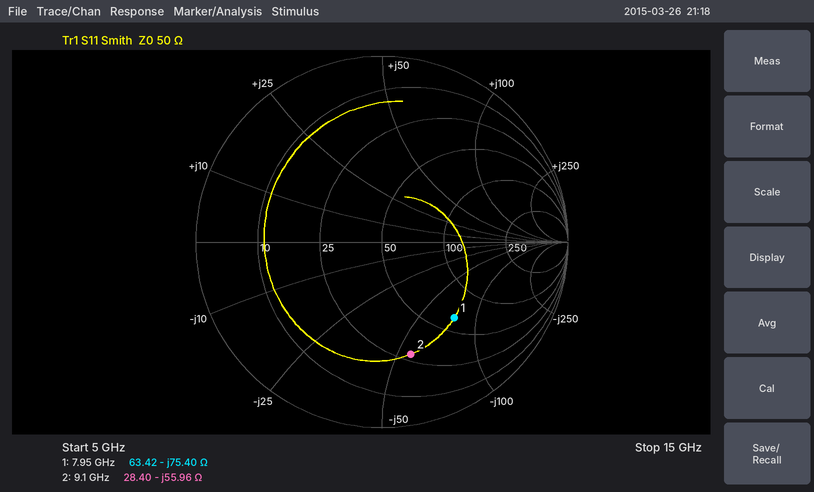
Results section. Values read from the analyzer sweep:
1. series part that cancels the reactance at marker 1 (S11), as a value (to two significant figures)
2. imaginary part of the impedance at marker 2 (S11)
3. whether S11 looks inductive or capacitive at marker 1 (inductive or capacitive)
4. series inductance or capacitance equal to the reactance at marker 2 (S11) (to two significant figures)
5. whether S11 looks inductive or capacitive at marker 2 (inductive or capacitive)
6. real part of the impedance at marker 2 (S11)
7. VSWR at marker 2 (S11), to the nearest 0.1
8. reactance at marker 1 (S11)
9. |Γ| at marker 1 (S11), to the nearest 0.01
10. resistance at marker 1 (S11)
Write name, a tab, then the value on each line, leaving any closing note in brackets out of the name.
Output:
series part that cancels the reactance at marker 1 (S11), as a value	1.5 nH
imaginary part of the impedance at marker 2	-55.96 Ω
whether S11 looks inductive or capacitive at marker 1	capacitive
series inductance or capacitance equal to the reactance at marker 2 (S11)	310 fF
whether S11 looks inductive or capacitive at marker 2	capacitive
real part of the impedance at marker 2	28.40 Ω
VSWR at marker 2 (S11), to the nearest 0.1	4.3
reactance at marker 1	-75.40 Ω
|Γ| at marker 1 (S11), to the nearest 0.01	0.56
resistance at marker 1	63.42 Ω
